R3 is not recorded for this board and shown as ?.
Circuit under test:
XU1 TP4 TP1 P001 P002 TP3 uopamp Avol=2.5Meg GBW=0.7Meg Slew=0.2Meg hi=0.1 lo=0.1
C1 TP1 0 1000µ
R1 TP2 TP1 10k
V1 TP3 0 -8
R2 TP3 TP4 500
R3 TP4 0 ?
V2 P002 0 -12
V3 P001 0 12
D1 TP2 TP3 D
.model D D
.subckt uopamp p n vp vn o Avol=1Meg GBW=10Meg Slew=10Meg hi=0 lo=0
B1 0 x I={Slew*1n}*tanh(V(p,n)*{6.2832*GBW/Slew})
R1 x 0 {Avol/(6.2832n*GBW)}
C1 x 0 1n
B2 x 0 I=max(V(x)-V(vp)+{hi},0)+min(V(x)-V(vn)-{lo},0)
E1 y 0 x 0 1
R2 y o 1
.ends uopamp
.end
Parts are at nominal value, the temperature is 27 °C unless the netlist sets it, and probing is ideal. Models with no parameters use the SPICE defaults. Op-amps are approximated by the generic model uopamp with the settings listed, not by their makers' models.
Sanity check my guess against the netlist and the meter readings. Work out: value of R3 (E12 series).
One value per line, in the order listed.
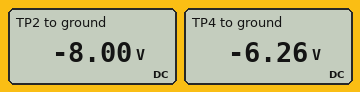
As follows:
1.8 kΩ
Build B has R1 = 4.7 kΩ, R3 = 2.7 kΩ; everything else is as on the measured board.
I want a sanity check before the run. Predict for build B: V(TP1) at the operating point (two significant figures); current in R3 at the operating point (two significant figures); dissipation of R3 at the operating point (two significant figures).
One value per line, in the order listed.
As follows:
-8.0 V
2.5 mA
17 mW
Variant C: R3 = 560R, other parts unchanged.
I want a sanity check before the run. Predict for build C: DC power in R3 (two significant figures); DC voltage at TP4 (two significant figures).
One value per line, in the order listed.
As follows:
32 mW
-4.2 V
